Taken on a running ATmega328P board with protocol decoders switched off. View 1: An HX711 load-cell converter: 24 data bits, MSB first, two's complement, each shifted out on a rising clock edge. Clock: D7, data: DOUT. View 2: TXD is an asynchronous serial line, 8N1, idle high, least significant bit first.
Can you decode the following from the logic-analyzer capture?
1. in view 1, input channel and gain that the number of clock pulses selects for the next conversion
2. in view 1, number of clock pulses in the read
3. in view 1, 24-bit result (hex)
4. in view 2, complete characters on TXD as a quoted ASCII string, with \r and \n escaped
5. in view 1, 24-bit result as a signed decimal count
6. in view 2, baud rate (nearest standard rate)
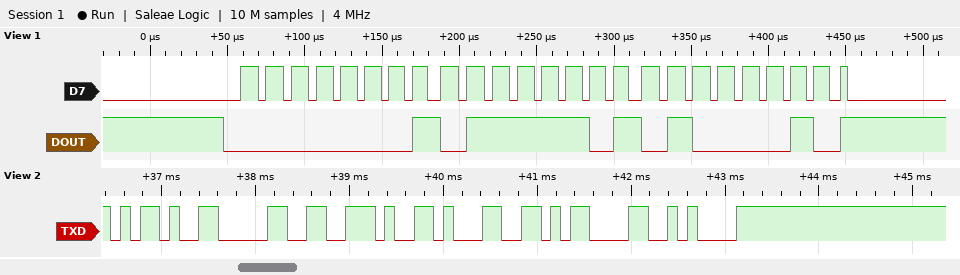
channel A, gain 128
25
0x017D42
"-0.1\r\n"
97602
9600 baud
